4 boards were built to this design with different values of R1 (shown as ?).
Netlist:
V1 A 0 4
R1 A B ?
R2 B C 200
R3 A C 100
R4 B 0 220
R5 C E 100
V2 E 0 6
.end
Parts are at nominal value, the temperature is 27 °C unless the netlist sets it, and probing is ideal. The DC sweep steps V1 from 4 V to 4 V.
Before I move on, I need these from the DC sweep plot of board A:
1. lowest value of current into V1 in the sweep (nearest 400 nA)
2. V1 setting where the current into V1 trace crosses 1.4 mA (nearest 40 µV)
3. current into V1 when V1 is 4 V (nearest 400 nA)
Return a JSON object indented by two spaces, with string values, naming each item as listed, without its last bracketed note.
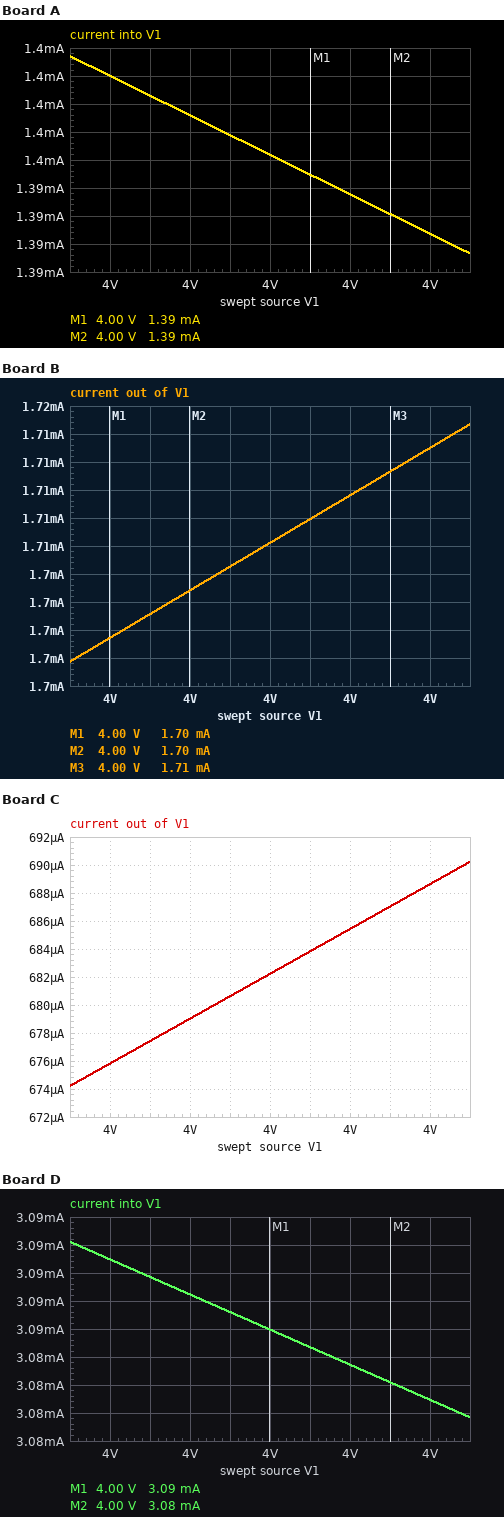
{
  "lowest value of current into V1 in the sweep": "1.3892 mA",
  "V1 setting where the current into V1 trace crosses 1.4 mA": "3.99948 V",
  "current into V1 when V1 is 4 V": "1.3908 mA"
}
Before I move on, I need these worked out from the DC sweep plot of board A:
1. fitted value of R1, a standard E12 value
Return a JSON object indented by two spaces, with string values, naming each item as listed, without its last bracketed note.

{
  "fitted value of R1, a standard E12 value": "270 Ω"
}
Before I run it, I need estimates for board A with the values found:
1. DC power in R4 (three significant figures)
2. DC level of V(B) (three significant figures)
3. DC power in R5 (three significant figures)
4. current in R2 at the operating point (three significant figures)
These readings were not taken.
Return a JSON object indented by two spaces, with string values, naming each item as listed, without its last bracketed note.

{
  "DC power in R4": "36.7 mW",
  "DC level of V(B)": "2.84 V",
  "DC power in R5": "20.5 mW",
  "current in R2 at the operating point": "8.63 mA"
}
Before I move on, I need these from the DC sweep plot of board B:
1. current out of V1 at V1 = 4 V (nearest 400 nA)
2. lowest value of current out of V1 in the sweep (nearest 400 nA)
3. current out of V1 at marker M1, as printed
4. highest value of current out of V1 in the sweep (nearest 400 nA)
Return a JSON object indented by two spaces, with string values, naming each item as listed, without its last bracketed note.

{
  "current out of V1 at V1 = 4 V": "1.7044 mA",
  "lowest value of current out of V1 in the sweep": "1.6976 mA",
  "current out of V1 at marker M1, as printed": "1.70 mA",
  "highest value of current out of V1 in the sweep": "1.7148 mA"
}
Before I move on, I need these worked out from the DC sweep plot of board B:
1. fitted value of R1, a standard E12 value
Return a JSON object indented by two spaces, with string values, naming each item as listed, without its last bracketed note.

{
  "fitted value of R1, a standard E12 value": "82 Ω"
}
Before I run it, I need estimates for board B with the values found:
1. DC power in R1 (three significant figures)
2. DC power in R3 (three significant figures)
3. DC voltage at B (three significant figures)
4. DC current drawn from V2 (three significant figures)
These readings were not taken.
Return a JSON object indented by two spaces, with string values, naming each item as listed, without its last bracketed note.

{
  "DC power in R1": "5.70 mW",
  "DC power in R3": "4.40 mW",
  "DC voltage at B": "3.32 V",
  "DC current drawn from V2": "13.4 mA"
}
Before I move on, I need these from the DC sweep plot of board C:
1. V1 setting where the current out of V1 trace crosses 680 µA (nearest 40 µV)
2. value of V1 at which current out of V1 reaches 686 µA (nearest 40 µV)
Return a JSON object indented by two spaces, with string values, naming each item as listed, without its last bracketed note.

{
  "V1 setting where the current out of V1 trace crosses 680 µA": "3.99972 V",
  "value of V1 at which current out of V1 reaches 686 µA": "4.00048 V"
}
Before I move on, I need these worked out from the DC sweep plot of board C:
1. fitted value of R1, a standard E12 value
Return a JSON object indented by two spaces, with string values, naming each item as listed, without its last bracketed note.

{
  "fitted value of R1, a standard E12 value": "120 Ω"
}
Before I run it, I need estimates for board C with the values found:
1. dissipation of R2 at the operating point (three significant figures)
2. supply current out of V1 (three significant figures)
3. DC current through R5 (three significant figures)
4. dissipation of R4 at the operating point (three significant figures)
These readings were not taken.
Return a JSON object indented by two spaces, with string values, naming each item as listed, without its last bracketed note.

{
  "dissipation of R2 at the operating point": "10.8 mW",
  "supply current out of V1": "682 µA",
  "DC current through R5": "13.7 mA",
  "dissipation of R4 at the operating point": "45.4 mW"
}
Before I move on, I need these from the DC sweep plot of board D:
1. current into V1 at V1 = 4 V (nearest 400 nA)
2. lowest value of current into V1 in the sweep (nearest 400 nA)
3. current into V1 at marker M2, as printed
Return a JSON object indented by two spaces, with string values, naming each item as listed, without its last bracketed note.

{
  "current into V1 at V1 = 4 V": "3.0872 mA",
  "lowest value of current into V1 in the sweep": "3.0796 mA",
  "current into V1 at marker M2, as printed": "3.08 mA"
}
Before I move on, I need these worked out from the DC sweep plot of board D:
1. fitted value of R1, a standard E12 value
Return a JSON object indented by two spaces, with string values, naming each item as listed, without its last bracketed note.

{
  "fitted value of R1, a standard E12 value": "680 Ω"
}
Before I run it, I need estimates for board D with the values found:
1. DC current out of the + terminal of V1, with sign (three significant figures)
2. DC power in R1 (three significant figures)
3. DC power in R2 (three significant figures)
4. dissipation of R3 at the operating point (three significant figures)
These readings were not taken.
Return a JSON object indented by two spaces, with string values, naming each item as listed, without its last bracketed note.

{
  "DC current out of the + terminal of V1, with sign": "-3.09 mA",
  "DC power in R1": "2.95 mW",
  "DC power in R2": "18.7 mW",
  "dissipation of R3 at the operating point": "2.67 mW"
}
